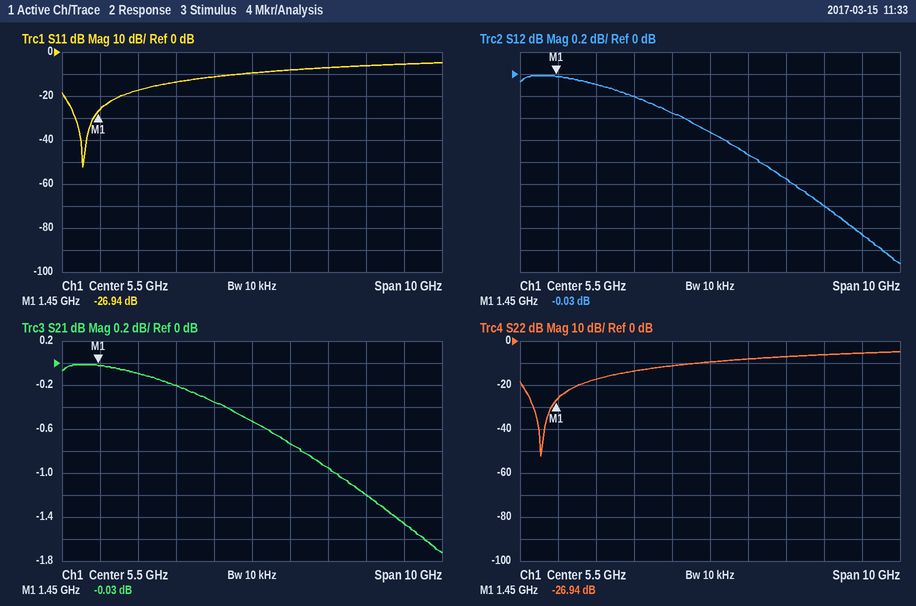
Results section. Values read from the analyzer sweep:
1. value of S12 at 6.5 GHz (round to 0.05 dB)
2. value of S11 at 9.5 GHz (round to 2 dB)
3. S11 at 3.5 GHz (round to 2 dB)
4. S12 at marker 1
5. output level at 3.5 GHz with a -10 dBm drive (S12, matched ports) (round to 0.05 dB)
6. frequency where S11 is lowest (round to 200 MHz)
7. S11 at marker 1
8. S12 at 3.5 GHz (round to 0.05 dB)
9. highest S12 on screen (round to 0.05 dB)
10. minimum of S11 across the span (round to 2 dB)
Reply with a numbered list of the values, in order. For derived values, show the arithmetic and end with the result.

1. -0.75 dB
2. -6 dB
3. -14 dB
4. -0.03 dB
5. -10 dBm + (-0.20 dB) = -10.20 dBm
6. 1.0 GHz
7. -26.94 dB
8. -0.20 dB
9. 0.00 dB
10. -52 dB
